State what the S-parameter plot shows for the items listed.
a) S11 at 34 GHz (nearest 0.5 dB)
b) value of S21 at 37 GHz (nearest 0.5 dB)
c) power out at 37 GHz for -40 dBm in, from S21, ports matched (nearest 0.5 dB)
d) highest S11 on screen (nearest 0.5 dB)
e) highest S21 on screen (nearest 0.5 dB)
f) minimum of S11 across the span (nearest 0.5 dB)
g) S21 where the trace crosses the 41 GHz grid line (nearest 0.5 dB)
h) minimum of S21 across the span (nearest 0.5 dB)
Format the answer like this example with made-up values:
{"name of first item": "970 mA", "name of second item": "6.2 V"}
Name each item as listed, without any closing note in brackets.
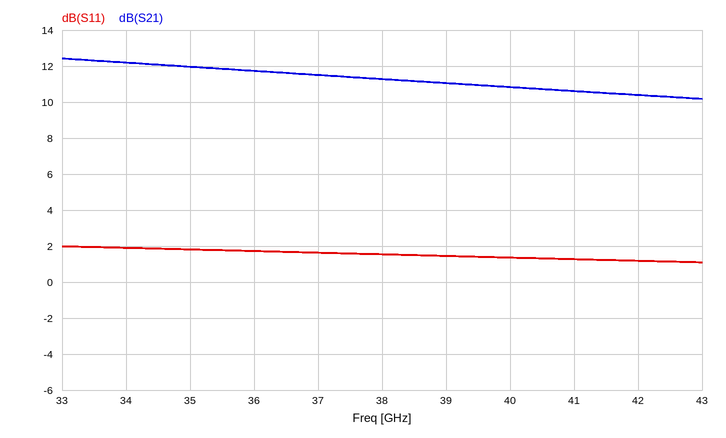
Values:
{"S11 at 34 GHz": "2.0 dB", "value of S21 at 37 GHz": "11.5 dB", "power out at 37 GHz for -40 dBm in, from S21, ports matched": "-28.5 dBm", "highest S11 on screen": "2.0 dB", "highest S21 on screen": "12.5 dB", "minimum of S11 across the span": "1.0 dB", "S21 where the trace crosses the 41 GHz grid line": "10.5 dB", "minimum of S21 across the span": "10.0 dB"}
